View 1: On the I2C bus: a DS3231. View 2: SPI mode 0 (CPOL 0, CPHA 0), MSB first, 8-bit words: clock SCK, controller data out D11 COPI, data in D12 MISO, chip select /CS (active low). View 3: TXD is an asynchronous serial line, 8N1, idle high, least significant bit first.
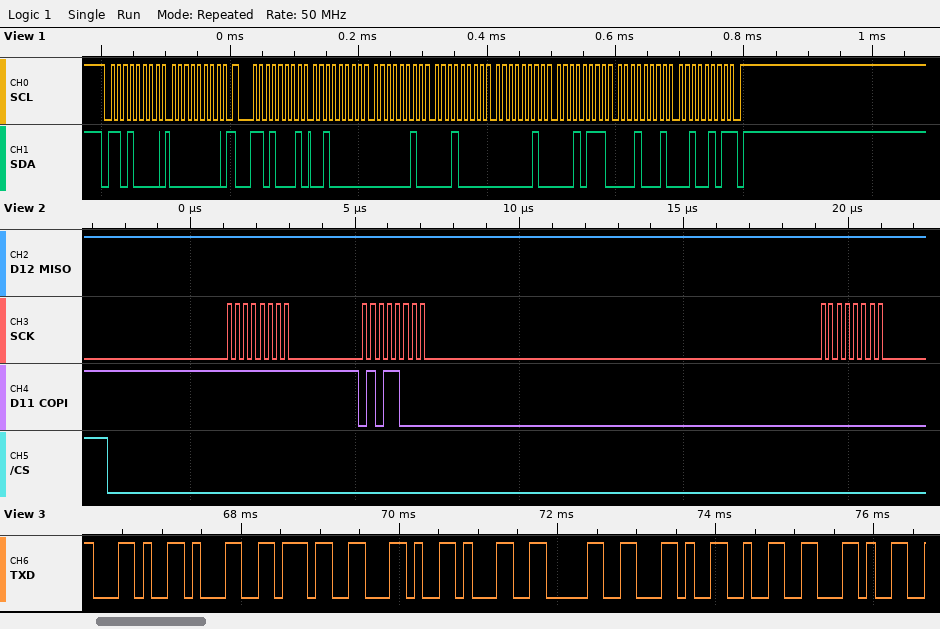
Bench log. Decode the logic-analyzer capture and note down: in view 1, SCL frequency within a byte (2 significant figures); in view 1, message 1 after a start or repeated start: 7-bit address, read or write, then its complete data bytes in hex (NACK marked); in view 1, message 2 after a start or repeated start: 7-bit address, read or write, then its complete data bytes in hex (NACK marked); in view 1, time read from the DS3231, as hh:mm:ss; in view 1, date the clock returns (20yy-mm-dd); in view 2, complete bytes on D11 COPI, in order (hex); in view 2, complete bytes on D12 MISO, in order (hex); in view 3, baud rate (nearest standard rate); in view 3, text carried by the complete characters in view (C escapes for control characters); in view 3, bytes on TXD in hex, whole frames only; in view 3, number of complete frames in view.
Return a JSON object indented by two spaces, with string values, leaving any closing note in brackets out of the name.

{
  "in view 1, SCL frequency within a byte": "100 kHz",
  "in view 1, message 1 after a start or repeated start: 7-bit address, read or write, then its complete data bytes in hex": "0x68 write: 00",
  "in view 1, message 2 after a start or repeated start: 7-bit address, read or write, then its complete data bytes in hex": "0x68 read: 20 02 10 02 17 11 25 NACK",
  "in view 1, time read from the DS3231, as hh:mm:ss": "10:02:20",
  "in view 1, date the clock returns": "2025-11-17",
  "in view 2, complete bytes on D11 COPI, in order": "0xFF 0x58 0x00",
  "in view 2, complete bytes on D12 MISO, in order": "0xFF 0xFF 0xFF",
  "in view 3, baud rate": "9600 baud",
  "in view 3, text carried by the complete characters in view": "\",17,10,2,\"",
  "in view 3, bytes on TXD in hex, whole frames only": "2C 31 37 2C 31 30 2C 32 2C",
  "in view 3, number of complete frames in view": "9"
}
